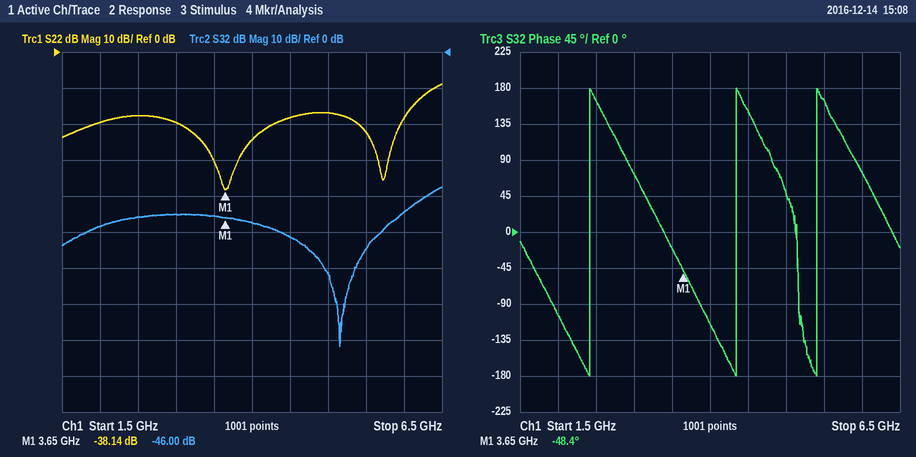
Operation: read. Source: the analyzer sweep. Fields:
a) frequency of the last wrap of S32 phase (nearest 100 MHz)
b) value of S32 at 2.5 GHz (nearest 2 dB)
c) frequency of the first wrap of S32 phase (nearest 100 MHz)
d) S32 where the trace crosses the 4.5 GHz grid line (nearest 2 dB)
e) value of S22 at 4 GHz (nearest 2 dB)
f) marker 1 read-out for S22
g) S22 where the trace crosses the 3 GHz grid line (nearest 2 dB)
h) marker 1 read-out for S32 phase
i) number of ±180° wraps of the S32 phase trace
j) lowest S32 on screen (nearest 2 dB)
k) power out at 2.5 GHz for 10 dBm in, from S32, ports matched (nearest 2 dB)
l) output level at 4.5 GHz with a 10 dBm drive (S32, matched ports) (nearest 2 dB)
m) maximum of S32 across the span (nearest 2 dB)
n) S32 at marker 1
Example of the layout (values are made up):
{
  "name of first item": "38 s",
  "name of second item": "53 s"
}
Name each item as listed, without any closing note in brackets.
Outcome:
{
  "frequency of the last wrap of S32 phase": "5.4 GHz",
  "value of S32 at 2.5 GHz": "-46 dB",
  "frequency of the first wrap of S32 phase": "2.4 GHz",
  "S32 where the trace crosses the 4.5 GHz grid line": "-52 dB",
  "value of S22 at 4 GHz": "-24 dB",
  "marker 1 read-out for S22": "-38.14 dB",
  "S22 where the trace crosses the 3 GHz grid line": "-20 dB",
  "marker 1 read-out for S32 phase": "-48.4°",
  "number of ±180° wraps of the S32 phase trace": "3",
  "lowest S32 on screen": "-82 dB",
  "power out at 2.5 GHz for 10 dBm in, from S32, ports matched": "-36 dBm",
  "output level at 4.5 GHz with a 10 dBm drive (S32, matched ports)": "-42 dBm",
  "maximum of S32 across the span": "-38 dB",
  "S32 at marker 1": "-46.00 dB"
}
